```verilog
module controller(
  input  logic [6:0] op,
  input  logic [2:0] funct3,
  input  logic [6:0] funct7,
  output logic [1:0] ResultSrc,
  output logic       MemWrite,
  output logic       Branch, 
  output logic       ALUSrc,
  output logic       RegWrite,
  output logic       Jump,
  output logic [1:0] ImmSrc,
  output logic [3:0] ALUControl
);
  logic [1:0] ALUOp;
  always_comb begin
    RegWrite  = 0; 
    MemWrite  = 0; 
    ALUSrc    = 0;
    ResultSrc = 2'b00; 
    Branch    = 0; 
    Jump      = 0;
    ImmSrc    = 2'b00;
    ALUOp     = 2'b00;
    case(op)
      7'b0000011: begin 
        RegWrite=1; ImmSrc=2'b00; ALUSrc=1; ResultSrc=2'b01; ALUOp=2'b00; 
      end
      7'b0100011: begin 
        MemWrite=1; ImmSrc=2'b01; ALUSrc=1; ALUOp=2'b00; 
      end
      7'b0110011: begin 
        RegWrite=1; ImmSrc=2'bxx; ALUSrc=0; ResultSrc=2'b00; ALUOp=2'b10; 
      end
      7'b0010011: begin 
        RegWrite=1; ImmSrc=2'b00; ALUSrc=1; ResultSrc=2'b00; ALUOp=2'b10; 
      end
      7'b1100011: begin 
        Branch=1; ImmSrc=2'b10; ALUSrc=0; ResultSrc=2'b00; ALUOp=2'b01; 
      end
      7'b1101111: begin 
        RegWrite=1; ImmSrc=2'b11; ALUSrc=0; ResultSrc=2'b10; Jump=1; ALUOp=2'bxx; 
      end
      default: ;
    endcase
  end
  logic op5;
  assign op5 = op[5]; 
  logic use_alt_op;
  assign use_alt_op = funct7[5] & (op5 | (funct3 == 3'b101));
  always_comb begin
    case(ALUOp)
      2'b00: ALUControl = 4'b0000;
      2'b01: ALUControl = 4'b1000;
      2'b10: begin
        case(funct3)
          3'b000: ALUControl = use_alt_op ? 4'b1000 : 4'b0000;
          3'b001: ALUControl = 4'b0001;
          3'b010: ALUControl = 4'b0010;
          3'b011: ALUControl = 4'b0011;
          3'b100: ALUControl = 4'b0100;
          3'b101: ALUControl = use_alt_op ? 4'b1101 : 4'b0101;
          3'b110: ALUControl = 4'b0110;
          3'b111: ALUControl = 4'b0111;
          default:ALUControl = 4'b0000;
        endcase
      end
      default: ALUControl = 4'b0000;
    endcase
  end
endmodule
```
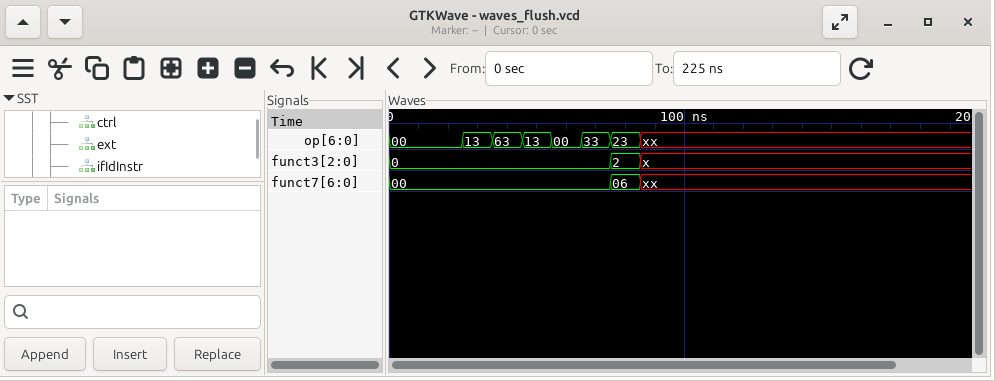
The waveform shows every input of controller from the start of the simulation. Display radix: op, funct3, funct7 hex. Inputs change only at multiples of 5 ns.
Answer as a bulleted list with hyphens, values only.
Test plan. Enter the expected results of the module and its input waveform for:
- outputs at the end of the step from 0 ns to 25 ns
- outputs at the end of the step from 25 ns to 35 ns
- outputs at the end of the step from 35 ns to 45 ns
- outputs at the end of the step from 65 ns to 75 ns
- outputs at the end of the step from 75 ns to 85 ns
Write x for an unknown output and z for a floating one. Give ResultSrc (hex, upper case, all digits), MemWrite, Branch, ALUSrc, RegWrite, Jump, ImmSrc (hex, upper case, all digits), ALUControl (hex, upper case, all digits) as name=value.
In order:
- ResultSrc=0, MemWrite=0, Branch=0, ALUSrc=0, RegWrite=0, Jump=0, ImmSrc=0, ALUControl=0
- ResultSrc=0, MemWrite=0, Branch=0, ALUSrc=1, RegWrite=1, Jump=0, ImmSrc=0, ALUControl=0
- ResultSrc=0, MemWrite=0, Branch=1, ALUSrc=0, RegWrite=0, Jump=0, ImmSrc=2, ALUControl=8
- ResultSrc=0, MemWrite=0, Branch=0, ALUSrc=0, RegWrite=1, Jump=0, ImmSrc=x, ALUControl=0
- ResultSrc=0, MemWrite=1, Branch=0, ALUSrc=1, RegWrite=0, Jump=0, ImmSrc=1, ALUControl=0
